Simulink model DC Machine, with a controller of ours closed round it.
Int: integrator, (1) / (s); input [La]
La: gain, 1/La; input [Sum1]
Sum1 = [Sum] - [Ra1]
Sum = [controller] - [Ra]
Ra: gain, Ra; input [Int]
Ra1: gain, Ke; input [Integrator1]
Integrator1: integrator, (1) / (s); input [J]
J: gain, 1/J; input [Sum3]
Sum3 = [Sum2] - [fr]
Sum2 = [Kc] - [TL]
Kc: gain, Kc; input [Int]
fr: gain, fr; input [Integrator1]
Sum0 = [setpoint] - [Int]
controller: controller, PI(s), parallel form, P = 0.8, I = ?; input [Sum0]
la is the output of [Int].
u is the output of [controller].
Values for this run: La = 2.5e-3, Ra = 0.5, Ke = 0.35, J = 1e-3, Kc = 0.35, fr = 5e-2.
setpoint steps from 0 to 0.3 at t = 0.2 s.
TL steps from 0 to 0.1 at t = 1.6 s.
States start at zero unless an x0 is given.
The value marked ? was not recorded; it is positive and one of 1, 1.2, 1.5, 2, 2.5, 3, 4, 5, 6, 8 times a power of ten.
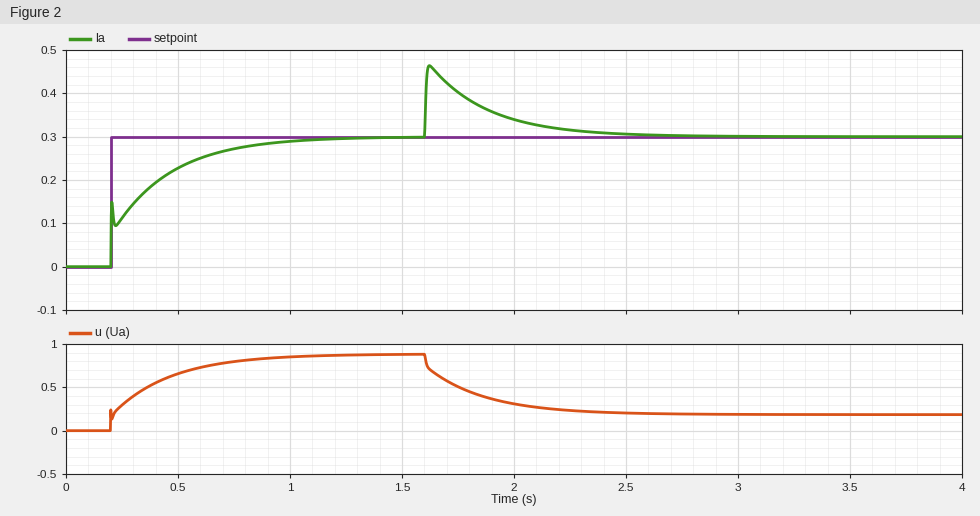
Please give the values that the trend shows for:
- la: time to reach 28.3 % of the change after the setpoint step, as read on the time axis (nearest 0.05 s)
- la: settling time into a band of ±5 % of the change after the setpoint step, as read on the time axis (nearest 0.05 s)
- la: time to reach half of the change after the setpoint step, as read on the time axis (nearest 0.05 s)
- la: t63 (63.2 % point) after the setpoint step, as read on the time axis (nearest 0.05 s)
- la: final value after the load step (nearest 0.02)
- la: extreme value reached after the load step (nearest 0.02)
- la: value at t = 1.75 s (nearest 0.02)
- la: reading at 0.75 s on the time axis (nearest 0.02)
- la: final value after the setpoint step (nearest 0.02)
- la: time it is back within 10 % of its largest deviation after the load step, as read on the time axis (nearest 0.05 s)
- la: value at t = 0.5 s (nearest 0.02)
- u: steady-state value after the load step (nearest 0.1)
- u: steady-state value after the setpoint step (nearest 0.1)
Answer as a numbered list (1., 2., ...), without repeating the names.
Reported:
1. 0.20 s
2. 0.90 s
3. 0.30 s
4. 0.40 s
5. 0.30
6. 0.46
7. 0.40
8. 0.28
9. 0.30
10. 2.25 s
11. 0.22
12. 0.2
13. 0.9
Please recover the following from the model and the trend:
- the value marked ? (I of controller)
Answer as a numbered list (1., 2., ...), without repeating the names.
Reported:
1. 15
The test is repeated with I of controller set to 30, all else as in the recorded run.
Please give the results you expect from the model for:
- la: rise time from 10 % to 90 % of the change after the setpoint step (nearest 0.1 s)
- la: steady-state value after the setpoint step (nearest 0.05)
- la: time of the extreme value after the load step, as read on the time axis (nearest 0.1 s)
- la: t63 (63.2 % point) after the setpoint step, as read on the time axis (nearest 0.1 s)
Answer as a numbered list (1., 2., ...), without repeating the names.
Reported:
1. 0.3 s
2. 0.30
3. 1.6 s
4. 0.3 s
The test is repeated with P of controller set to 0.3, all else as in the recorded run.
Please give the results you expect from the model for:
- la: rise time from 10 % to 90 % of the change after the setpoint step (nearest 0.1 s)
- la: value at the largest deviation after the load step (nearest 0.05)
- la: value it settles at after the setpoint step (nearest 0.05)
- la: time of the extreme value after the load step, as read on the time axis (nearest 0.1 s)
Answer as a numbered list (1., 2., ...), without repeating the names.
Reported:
1. 0.5 s
2. 0.50
3. 0.30
4. 1.6 s
